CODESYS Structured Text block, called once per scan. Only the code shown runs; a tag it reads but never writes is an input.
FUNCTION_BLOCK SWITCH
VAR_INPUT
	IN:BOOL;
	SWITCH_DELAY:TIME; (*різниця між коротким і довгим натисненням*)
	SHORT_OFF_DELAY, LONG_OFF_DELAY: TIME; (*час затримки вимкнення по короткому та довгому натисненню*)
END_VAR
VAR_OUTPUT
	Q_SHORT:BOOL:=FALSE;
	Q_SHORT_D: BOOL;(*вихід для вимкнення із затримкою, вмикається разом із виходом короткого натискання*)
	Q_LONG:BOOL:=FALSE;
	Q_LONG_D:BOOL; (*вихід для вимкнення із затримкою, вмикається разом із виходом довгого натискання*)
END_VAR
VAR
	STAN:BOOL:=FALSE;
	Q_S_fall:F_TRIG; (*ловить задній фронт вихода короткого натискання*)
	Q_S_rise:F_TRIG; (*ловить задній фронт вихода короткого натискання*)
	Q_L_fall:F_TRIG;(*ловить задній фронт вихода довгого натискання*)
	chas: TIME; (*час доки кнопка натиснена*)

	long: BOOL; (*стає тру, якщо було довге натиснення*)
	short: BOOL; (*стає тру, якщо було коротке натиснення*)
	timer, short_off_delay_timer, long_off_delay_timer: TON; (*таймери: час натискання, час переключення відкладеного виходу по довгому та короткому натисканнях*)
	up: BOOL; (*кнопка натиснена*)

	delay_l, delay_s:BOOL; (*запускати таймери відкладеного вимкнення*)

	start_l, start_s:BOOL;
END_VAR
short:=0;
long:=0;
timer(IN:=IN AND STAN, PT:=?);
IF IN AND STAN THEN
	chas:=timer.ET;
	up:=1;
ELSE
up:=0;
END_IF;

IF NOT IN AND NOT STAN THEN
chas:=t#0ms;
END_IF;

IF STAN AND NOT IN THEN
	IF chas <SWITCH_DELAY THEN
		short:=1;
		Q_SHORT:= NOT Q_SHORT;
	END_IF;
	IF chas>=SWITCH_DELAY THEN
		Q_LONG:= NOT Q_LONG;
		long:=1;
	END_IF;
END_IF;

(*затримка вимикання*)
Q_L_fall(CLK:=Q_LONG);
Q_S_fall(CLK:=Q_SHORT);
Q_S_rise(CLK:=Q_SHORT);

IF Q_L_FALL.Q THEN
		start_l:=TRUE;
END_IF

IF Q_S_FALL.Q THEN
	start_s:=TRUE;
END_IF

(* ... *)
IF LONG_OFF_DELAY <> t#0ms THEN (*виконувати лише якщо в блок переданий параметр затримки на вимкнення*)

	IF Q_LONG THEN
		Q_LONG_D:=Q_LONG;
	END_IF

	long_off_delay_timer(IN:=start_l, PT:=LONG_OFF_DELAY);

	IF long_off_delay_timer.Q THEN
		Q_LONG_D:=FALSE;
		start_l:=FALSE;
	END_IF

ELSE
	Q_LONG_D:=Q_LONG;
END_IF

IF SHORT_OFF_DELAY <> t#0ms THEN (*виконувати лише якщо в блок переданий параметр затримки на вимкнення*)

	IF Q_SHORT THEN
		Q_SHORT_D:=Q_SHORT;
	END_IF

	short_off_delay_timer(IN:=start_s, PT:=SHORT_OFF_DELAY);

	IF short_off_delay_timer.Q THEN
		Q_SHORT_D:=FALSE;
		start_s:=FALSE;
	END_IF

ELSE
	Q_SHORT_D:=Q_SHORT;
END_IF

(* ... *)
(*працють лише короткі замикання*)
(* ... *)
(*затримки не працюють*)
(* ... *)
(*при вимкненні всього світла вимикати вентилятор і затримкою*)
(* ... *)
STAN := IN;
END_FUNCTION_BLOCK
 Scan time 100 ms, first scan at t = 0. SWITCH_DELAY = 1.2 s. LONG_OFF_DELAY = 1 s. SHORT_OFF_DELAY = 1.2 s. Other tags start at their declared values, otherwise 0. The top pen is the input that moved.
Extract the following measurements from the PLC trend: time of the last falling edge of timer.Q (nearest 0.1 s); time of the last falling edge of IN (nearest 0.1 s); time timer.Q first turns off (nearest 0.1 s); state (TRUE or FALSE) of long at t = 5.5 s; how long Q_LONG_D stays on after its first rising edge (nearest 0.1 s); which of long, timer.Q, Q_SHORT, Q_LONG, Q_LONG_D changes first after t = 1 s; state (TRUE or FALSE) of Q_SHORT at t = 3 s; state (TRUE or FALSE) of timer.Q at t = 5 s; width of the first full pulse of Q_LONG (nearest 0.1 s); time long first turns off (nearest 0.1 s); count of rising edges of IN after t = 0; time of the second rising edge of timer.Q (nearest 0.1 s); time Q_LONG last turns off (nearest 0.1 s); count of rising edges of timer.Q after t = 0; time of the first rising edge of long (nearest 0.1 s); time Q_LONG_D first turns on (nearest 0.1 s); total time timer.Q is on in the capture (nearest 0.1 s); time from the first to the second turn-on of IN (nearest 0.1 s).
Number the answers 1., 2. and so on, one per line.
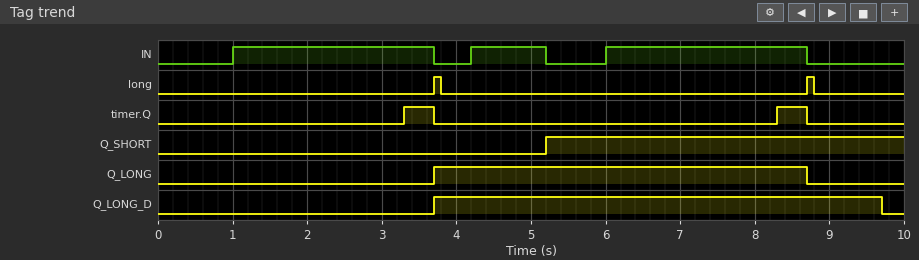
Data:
1. 8.7 s
2. 8.7 s
3. 3.7 s
4. FALSE
5. 6.0 s
6. timer.Q
7. FALSE
8. FALSE
9. 5.0 s
10. 3.8 s
11. 3
12. 8.3 s
13. 8.7 s
14. 2
15. 3.7 s
16. 3.7 s
17. 0.8 s
18. 3.2 s
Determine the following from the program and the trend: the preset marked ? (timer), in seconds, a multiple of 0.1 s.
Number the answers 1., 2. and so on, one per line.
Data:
1. 2.2 s
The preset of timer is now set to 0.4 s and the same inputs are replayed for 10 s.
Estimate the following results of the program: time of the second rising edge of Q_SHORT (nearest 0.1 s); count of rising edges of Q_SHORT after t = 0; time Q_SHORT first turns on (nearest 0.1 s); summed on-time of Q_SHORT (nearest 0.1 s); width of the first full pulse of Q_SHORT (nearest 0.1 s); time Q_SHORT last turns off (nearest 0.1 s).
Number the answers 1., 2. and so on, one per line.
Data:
1. 8.7 s
2. 2
3. 3.7 s
4. 2.8 s
5. 1.5 s
6. 5.2 s
